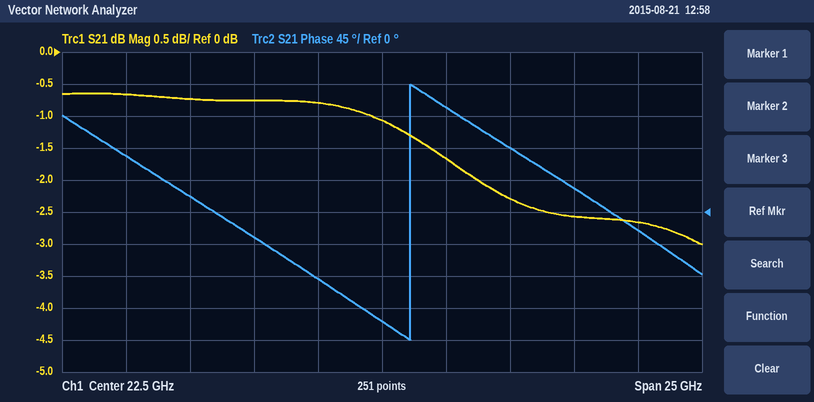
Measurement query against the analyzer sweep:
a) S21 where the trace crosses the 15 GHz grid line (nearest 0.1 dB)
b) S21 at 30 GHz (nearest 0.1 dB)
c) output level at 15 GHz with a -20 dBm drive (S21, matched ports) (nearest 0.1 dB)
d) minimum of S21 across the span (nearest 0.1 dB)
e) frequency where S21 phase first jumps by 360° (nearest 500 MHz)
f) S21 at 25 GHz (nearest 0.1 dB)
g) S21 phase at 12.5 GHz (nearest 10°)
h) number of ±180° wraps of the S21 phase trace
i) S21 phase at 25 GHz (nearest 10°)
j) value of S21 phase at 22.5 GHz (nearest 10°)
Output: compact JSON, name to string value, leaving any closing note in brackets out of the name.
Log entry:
{"S21 where the trace crosses the 15 GHz grid line": "-0.7 dB", "S21 at 30 GHz": "-2.6 dB", "output level at 15 GHz with a -20 dBm drive (S21, matched ports)": "-20.7 dBm", "minimum of S21 across the span": "-3.0 dB", "frequency where S21 phase first jumps by 360°": "23.5 GHz", "S21 at 25 GHz": "-1.7 dB", "S21 phase at 12.5 GHz": "80°", "number of ±180° wraps of the S21 phase trace": "1", "S21 phase at 25 GHz": "150°", "value of S21 phase at 22.5 GHz": "-150°"}
